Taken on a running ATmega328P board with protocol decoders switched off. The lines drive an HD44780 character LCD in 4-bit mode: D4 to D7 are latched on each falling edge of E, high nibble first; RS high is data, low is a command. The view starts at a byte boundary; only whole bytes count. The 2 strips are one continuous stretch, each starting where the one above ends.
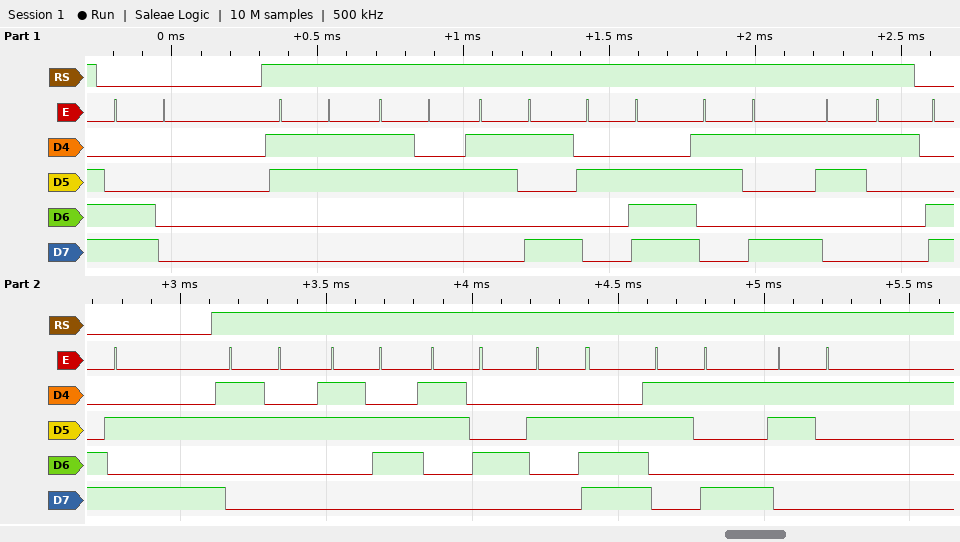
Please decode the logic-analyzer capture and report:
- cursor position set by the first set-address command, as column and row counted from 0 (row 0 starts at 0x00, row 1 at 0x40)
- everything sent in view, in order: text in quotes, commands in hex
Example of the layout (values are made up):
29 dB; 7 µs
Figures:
column 0, row 1; 0xC0 "329.91" 0xCA "264.91"
